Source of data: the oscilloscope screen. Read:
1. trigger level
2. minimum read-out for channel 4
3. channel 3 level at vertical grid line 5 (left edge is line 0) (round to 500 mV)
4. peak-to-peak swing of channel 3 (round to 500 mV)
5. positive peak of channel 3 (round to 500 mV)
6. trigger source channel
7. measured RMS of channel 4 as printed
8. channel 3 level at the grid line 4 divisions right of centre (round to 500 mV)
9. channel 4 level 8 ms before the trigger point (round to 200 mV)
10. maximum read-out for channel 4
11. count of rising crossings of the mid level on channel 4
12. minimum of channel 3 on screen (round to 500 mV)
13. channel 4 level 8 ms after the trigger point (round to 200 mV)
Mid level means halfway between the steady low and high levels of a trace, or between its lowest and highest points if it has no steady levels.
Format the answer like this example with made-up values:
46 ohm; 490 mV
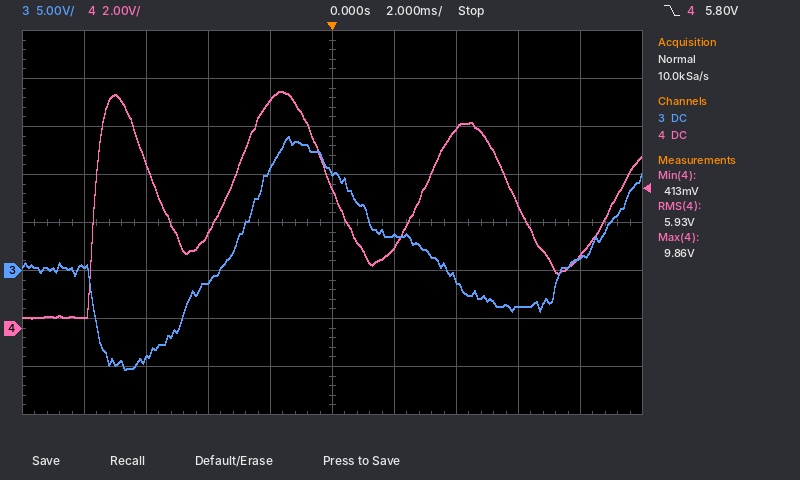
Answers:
5.80 V; 413 mV; 10.5 V; 24.5 V; 14.0 V; channel 4; 5.93 V; 1.5 V; 400 mV; 9.86 V; 4; -10.5 V; 3.0 V
